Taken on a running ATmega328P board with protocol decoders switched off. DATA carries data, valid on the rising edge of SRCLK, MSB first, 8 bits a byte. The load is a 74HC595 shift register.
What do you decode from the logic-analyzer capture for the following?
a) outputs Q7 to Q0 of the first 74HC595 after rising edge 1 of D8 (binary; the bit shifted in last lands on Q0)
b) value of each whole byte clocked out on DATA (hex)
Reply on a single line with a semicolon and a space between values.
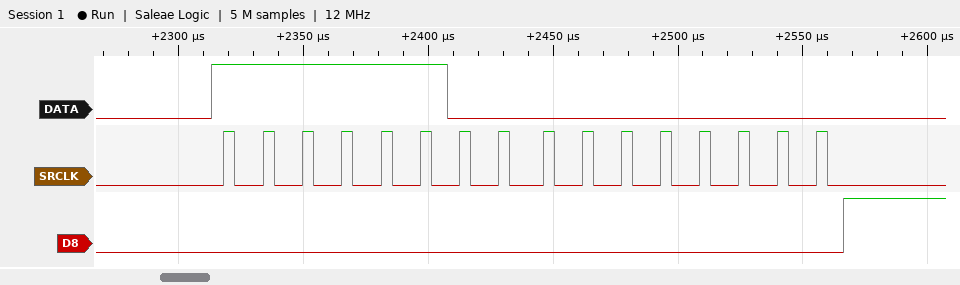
00000000; FC 00
